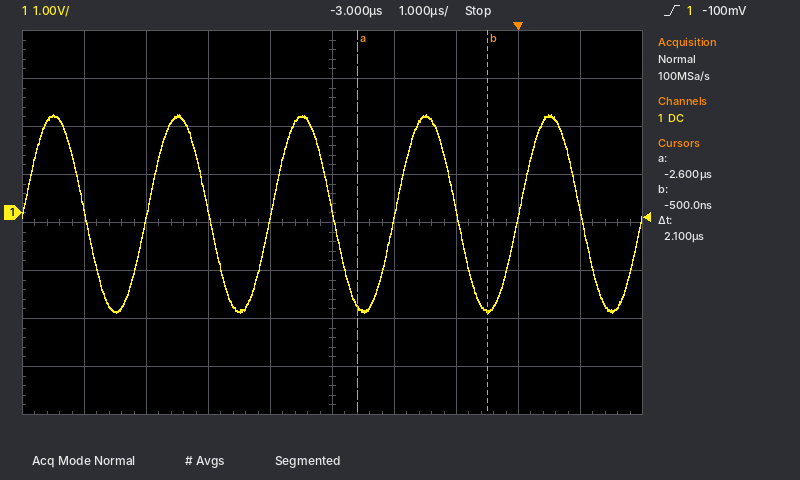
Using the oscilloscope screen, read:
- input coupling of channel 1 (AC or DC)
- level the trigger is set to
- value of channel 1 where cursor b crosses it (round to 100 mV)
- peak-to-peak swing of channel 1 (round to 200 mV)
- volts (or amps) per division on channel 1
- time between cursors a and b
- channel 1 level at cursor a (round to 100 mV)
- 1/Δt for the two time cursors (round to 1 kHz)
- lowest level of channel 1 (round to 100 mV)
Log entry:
DC
-100 mV
-2.0 V
4.2 V
1 V
2.1 µs
-1.9 V
476 kHz
-2.1 V
